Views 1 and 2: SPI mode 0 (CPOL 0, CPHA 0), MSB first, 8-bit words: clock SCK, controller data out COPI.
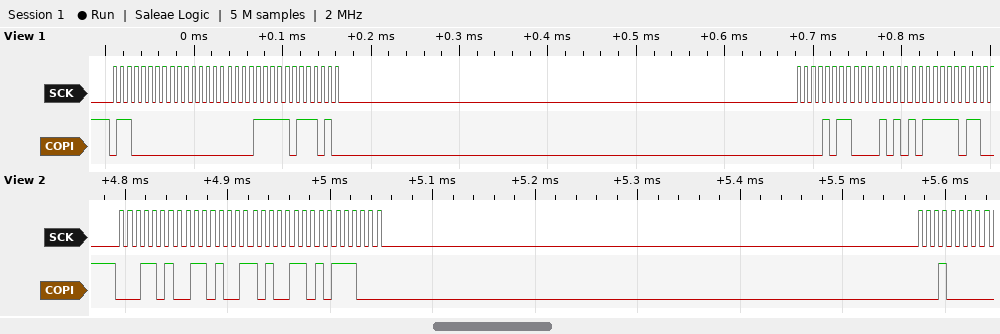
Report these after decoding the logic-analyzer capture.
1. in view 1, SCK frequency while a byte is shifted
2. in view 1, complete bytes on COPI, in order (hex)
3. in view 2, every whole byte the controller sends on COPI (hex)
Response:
125 kHz
60 00 0F BA 0B 0A BE
0x1A 0x69 0xA6 0xB8 0x10
